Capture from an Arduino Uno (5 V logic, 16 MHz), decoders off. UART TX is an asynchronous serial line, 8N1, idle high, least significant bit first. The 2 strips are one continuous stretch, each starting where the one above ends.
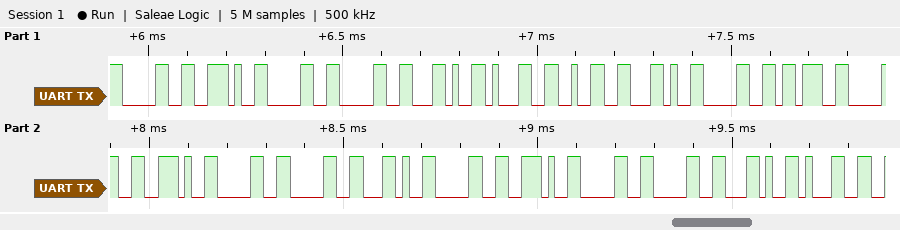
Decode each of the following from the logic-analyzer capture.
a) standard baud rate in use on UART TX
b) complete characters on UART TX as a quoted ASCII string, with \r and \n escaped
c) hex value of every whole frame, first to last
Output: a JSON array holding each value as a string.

["57600 baud", "\"0.00,12,0;0.00,0.00,1\"", "30 2E 30 30 2C 31 32 2C 30 3B 30 2E 30 30 2C 30 2E 30 30 2C 31"]
